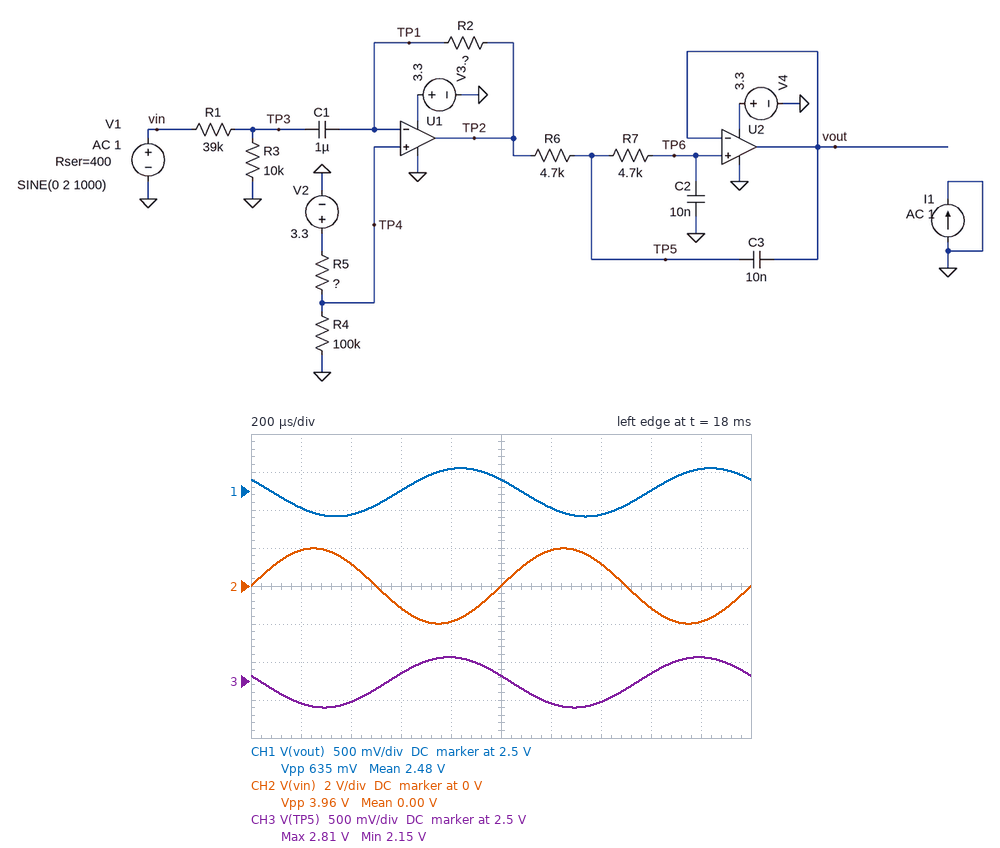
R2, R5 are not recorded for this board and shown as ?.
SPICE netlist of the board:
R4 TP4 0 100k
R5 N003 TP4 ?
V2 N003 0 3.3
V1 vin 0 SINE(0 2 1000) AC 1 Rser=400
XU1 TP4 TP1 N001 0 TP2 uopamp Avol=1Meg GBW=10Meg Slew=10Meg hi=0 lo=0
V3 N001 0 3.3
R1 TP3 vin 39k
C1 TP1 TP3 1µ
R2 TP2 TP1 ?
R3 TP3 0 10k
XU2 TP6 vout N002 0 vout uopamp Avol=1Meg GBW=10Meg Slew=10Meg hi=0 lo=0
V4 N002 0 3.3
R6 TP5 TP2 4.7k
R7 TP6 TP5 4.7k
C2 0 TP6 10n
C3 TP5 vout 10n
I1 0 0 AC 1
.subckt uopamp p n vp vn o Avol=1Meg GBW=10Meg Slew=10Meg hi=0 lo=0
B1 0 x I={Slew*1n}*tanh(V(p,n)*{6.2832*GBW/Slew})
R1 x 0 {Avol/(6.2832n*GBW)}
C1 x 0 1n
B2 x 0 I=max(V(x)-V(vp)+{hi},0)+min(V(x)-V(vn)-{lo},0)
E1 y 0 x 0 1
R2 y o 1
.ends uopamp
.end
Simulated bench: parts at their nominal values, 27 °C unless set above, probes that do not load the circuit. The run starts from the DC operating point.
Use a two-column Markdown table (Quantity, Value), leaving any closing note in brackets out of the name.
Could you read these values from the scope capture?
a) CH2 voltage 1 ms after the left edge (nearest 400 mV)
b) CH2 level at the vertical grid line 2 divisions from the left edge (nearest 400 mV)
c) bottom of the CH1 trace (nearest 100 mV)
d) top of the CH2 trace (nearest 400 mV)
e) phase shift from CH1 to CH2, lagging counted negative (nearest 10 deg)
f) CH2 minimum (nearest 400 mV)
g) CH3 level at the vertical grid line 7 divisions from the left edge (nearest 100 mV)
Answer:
| Quantity | Value |
|---|---|
| CH2 voltage 1 ms after the left edge | 0 V |
| CH2 level at the vertical grid line 2 divisions from the left edge | 1.2 V |
| bottom of the CH1 trace | 2.2 V |
| top of the CH2 trace | 2.0 V |
| phase shift from CH1 to CH2, lagging counted negative | -150 deg |
| CH2 minimum | -2.0 V |
| CH3 level at the vertical grid line 7 divisions from the left edge | 2.2 V |
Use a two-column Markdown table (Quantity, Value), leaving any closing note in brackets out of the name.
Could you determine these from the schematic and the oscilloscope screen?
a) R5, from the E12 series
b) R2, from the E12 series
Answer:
| Quantity | Value |
|---|---|
| R5, from the E12 series | 33 kΩ |
| R2, from the E12 series | 6.8 kΩ |
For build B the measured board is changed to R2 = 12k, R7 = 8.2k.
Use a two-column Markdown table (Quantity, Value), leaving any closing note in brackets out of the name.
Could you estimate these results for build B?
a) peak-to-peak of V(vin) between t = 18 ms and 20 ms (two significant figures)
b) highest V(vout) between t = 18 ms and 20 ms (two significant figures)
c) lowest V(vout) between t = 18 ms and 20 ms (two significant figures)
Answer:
| Quantity | Value |
|---|---|
| peak-to-peak of V(vin) between t = 18 ms and 20 ms | 4.0 V |
| highest V(vout) between t = 18 ms and 20 ms | 3.0 V |
| lowest V(vout) between t = 18 ms and 20 ms | 2.0 V |
